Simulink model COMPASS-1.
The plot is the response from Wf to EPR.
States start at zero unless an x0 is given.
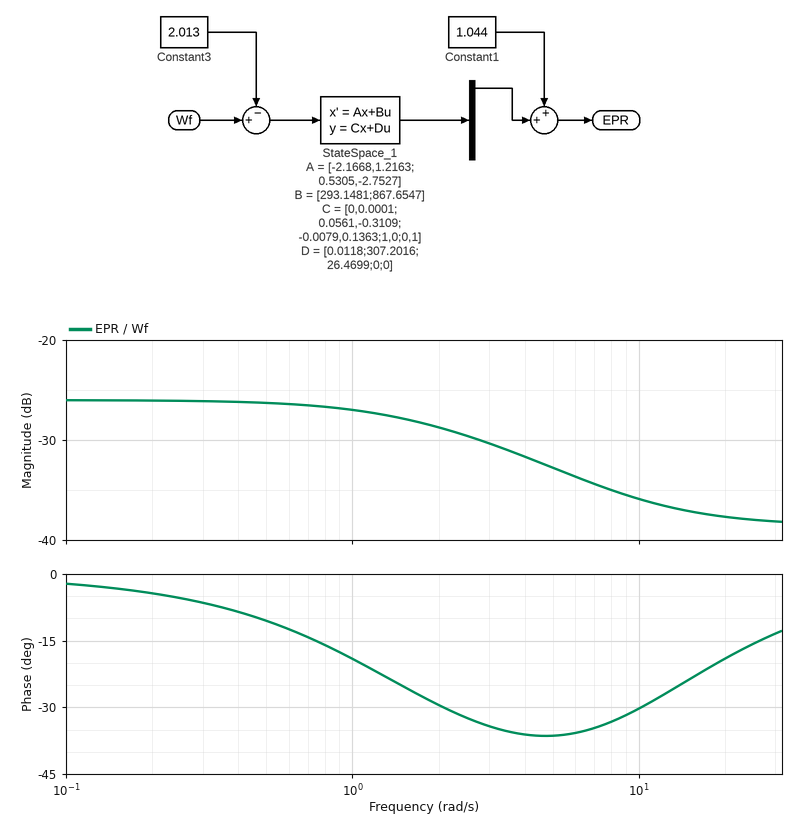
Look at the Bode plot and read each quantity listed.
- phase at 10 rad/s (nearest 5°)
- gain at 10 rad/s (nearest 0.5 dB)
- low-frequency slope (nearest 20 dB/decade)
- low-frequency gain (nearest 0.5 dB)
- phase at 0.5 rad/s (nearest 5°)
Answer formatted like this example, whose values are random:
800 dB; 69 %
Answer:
-30°; -36.0 dB; 0 dB/decade; -26.0 dB; -10°
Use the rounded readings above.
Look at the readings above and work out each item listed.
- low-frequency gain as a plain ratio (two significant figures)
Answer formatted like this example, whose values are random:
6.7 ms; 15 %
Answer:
0.050
